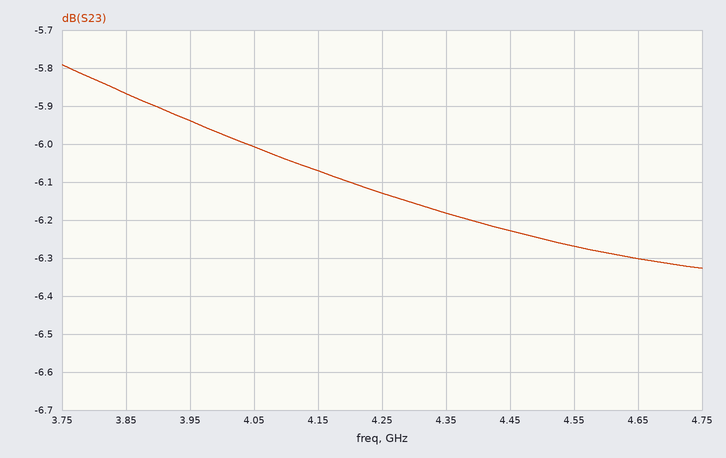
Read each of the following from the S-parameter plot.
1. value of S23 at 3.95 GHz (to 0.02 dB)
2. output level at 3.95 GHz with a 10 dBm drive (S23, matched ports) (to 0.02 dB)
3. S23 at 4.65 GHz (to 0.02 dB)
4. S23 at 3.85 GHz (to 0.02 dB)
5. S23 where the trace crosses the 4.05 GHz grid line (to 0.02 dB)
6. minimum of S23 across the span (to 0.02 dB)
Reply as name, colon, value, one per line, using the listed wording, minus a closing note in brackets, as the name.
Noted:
value of S23 at 3.95 GHz: -5.94 dB
output level at 3.95 GHz with a 10 dBm drive (S23, matched ports): 4.06 dBm
S23 at 4.65 GHz: -6.30 dB
S23 at 3.85 GHz: -5.86 dB
S23 where the trace crosses the 4.05 GHz grid line: -6.00 dB
minimum of S23 across the span: -6.32 dB
